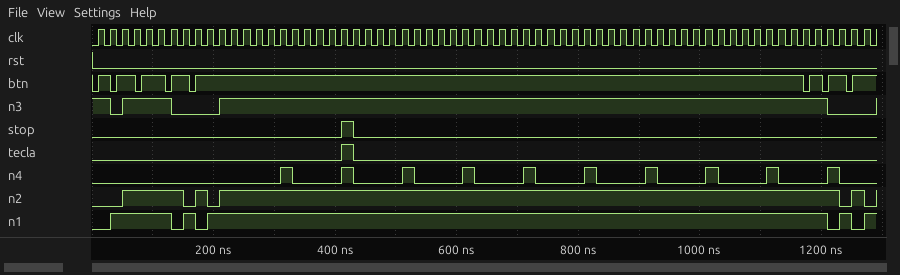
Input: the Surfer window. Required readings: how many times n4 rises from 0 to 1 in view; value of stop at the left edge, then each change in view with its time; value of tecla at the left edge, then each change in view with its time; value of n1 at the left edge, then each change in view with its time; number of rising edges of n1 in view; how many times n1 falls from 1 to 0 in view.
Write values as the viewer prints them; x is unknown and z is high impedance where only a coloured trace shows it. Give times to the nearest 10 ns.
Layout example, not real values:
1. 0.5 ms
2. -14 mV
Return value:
1. 10
2. 0, 1 at 410 ns, 0 at 430 ns
3. 0, 1 at 410 ns, 0 at 430 ns
4. 0, 1 at 30 ns, 0 at 130 ns, 1 at 150 ns, 0 at 170 ns, 1 at 190 ns, 0 at 1210 ns, 1 at 1230 ns, 0 at 1250 ns, 1 at 1270 ns
5. 5
6. 4
